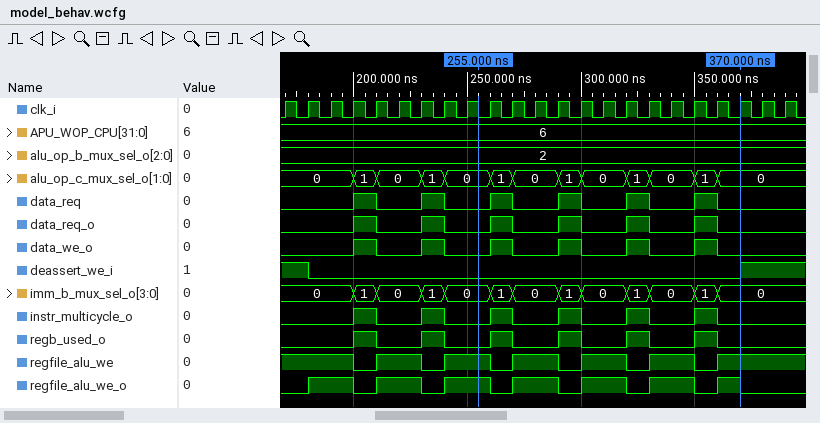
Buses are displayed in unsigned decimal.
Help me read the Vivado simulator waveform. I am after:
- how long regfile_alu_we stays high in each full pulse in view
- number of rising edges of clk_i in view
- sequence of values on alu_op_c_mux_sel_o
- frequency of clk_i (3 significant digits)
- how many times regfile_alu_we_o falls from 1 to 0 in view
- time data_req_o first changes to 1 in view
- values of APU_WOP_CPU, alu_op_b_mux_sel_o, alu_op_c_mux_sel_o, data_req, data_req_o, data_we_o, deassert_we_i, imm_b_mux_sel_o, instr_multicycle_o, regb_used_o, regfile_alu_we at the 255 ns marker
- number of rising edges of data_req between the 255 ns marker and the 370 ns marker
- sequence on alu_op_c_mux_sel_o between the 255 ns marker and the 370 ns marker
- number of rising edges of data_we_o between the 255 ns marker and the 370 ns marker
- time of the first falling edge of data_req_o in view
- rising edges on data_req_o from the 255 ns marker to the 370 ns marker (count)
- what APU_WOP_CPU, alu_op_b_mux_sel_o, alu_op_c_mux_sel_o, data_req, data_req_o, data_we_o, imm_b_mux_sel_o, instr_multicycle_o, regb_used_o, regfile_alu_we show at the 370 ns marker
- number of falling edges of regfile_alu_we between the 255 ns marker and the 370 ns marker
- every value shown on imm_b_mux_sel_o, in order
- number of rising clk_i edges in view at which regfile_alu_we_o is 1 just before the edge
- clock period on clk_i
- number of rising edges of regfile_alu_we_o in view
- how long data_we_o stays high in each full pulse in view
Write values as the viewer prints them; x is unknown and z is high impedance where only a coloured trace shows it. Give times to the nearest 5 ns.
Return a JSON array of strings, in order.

["20 ns, 20 ns, 20 ns, 20 ns, 20 ns", "23", "0, 1, 0, 1, 0, 1, 0, 1, 0, 1, 0, 1, 0", "100 MHz", "7", "200 ns", "APU_WOP_CPU=6, alu_op_b_mux_sel_o=2, alu_op_c_mux_sel_o=0, data_req=0, data_req_o=0, data_we_o=0, deassert_we_i=0, imm_b_mux_sel_o=0, instr_multicycle_o=0, regb_used_o=0, regfile_alu_we=1", "4", "0, 1, 0, 1, 0, 1, 0, 1, 0", "4", "210 ns", "4", "APU_WOP_CPU=6, alu_op_b_mux_sel_o=2, alu_op_c_mux_sel_o=0, data_req=0, data_req_o=0, data_we_o=0, imm_b_mux_sel_o=0, instr_multicycle_o=0, regb_used_o=0, regfile_alu_we=1", "4", "0, 1, 0, 1, 0, 1, 0, 1, 0, 1, 0, 1, 0", "13", "10 ns", "7", "10 ns, 10 ns, 10 ns, 10 ns, 10 ns, 10 ns"]
